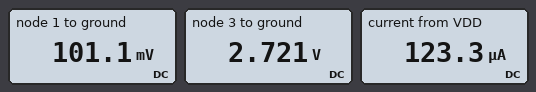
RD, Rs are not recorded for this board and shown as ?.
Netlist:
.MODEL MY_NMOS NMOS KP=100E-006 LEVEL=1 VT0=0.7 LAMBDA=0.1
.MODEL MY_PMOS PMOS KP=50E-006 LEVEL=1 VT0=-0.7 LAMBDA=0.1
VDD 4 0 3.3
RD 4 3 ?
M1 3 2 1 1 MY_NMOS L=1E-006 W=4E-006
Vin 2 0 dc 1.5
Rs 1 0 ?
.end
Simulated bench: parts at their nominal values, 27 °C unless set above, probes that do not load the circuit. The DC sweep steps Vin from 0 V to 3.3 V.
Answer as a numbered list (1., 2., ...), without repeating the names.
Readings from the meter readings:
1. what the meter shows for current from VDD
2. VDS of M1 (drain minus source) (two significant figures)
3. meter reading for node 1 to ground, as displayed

1. 123.3 µA
2. 2.6 V
3. 101.1 mV
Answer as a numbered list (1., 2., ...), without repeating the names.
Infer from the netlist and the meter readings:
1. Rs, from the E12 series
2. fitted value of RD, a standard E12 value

1. 820 Ω
2. 4.7 kΩ
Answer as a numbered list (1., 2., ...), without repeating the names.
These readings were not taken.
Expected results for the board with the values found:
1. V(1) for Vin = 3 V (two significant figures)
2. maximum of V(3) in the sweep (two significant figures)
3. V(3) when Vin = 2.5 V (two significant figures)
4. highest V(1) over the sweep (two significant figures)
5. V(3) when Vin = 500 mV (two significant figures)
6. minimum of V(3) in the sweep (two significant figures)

1. 390 mV
2. 3.3 V
3. 1.3 V
4. 400 mV
5. 3.3 V
6. 1.0 V
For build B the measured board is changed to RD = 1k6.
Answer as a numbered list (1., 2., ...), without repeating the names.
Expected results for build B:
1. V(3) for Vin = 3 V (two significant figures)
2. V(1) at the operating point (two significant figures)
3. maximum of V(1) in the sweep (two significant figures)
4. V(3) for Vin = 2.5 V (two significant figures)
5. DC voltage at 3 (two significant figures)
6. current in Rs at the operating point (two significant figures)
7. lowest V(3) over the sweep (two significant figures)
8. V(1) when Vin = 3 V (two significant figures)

1. 2.2 V
2. 100 mV
3. 650 mV
4. 2.5 V
5. 3.1 V
6. 130 µA
7. 2.0 V
8. 570 mV
